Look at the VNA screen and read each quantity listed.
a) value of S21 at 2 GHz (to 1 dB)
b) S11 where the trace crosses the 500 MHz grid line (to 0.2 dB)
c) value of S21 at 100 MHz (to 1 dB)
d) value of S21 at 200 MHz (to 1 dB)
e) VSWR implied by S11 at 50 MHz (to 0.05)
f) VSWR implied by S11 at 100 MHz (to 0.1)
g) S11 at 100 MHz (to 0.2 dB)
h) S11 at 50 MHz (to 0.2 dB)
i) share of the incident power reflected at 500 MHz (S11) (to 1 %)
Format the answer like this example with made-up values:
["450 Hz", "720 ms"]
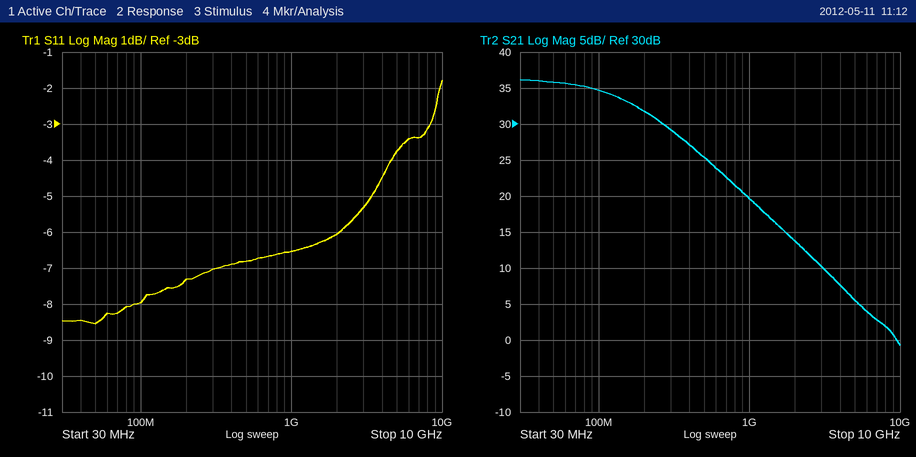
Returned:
["14 dB", "-6.8 dB", "35 dB", "32 dB", "2.20", "2.3", "-8.0 dB", "-8.6 dB", "21 %"]
